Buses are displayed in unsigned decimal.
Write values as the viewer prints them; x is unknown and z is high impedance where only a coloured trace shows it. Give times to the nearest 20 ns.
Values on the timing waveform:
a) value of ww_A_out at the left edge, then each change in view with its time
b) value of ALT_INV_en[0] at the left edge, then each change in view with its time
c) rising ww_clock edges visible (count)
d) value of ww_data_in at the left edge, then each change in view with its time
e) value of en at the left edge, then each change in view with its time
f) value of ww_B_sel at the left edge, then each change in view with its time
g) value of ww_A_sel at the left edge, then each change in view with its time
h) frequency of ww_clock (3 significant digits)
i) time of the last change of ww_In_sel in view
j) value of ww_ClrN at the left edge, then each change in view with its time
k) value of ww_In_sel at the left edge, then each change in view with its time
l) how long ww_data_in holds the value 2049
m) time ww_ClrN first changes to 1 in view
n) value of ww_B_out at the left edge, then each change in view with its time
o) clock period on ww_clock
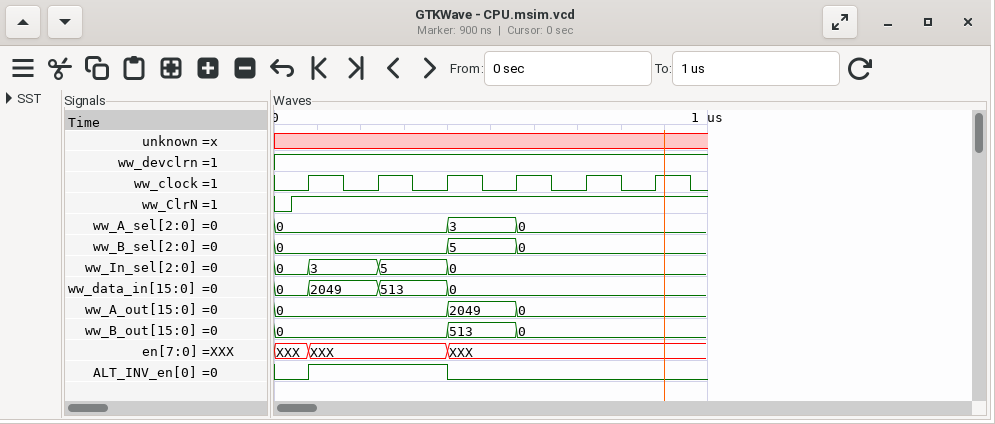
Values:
0, 2049 at 400 ns, 0 at 560 ns
0, 1 at 80 ns, 0 at 400 ns
6
0, 2049 at 80 ns, 513 at 240 ns, 0 at 400 ns
XXX, XXX at 80 ns, XXX at 400 ns
0, 5 at 400 ns, 0 at 560 ns
0, 3 at 400 ns, 0 at 560 ns
6.25 MHz
400 ns
0, 1 at 40 ns
0, 3 at 80 ns, 5 at 240 ns, 0 at 400 ns
160 ns
40 ns
0, 513 at 400 ns, 0 at 560 ns
160 ns
